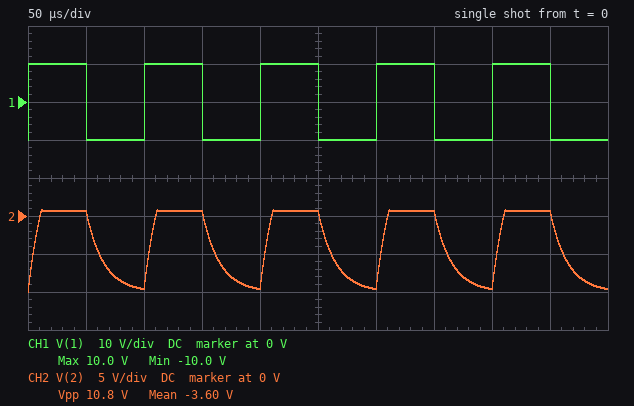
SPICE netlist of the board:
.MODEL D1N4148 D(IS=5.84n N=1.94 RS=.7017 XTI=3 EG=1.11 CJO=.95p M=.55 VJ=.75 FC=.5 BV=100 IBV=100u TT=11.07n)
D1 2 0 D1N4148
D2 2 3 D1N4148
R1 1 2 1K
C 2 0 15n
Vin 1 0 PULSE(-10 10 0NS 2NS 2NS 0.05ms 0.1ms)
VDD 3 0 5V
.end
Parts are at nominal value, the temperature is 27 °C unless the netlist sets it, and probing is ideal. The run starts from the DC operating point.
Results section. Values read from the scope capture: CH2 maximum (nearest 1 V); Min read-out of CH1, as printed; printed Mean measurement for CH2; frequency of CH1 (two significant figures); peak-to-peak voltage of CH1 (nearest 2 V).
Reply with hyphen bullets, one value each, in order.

- 1 V
- -10.0 V
- -3.60 V
- 10 kHz
- 20 V
